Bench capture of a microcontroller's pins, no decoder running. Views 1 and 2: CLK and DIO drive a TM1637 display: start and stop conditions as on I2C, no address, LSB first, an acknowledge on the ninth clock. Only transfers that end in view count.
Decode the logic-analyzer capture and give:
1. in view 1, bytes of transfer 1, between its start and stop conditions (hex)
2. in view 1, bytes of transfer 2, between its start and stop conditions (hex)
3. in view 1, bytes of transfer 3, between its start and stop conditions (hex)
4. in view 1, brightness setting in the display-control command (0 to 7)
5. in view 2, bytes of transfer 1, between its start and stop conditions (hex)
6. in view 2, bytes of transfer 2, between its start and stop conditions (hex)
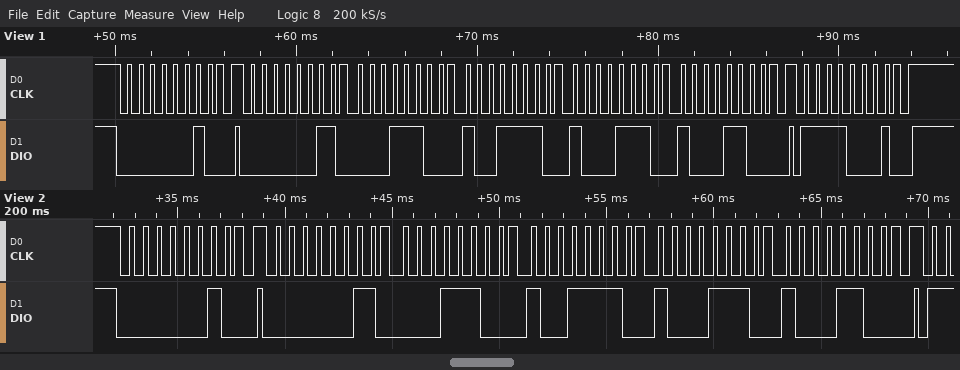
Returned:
40
C0 38 79 71 31
8F
7
40
C0 38 79 71 31
